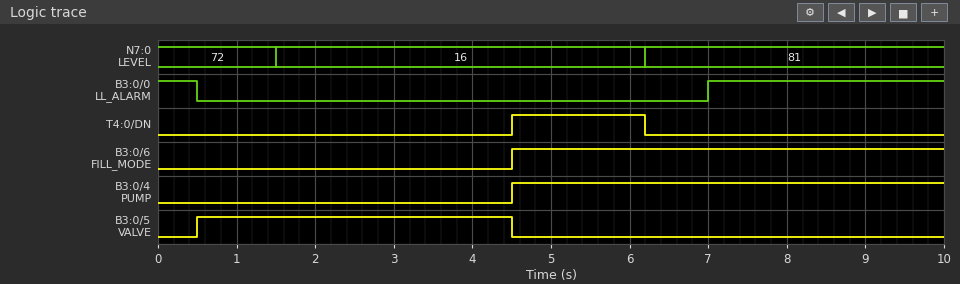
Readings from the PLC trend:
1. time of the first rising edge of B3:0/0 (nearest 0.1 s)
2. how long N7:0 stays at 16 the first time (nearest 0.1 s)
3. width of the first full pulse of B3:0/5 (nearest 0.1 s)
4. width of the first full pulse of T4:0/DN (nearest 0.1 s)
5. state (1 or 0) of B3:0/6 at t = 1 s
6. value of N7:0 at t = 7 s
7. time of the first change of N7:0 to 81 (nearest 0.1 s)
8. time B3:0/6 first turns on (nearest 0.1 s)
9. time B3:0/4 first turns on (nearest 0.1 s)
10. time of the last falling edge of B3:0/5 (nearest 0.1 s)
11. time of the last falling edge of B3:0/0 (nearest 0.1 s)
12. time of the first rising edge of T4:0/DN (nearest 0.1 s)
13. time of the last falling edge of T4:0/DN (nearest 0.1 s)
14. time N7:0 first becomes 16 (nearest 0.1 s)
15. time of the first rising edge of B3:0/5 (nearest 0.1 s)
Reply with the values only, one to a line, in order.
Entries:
7.0 s
4.7 s
4.0 s
1.7 s
0
81
6.2 s
4.5 s
4.5 s
4.5 s
0.5 s
4.5 s
6.2 s
1.5 s
0.5 s
